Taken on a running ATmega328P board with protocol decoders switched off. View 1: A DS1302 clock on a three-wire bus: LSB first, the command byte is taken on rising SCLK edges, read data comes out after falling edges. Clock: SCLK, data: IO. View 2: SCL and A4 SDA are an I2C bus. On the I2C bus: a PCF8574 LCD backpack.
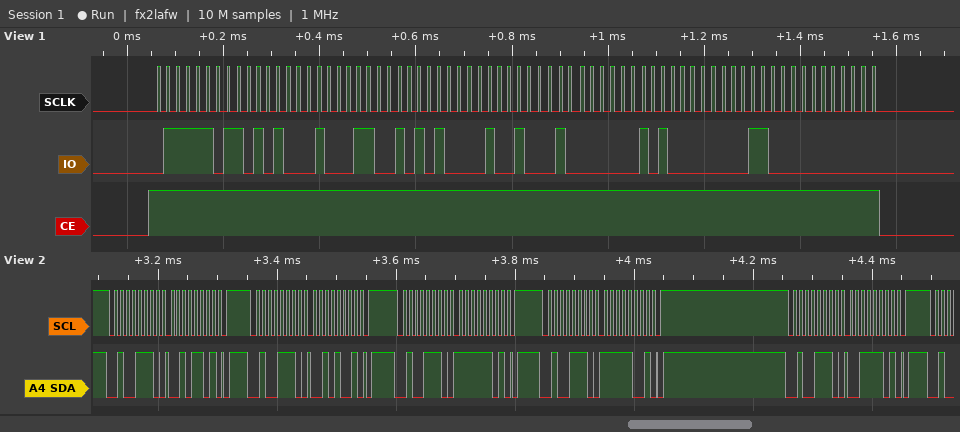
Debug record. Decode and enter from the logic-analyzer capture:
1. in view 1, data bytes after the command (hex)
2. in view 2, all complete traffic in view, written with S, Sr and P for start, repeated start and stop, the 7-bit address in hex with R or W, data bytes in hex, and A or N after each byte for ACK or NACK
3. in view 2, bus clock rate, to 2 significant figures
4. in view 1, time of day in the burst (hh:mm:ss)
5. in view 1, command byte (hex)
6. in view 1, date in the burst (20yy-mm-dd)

15 31 15 12 01 05 18 00
S 27W A 2D A P S 27W A 29 A P S 27W A FD A P S 27W A F9 A P S 27W A 3D A P
100 kHz
15:31:15
0xBE
2018-01-12
